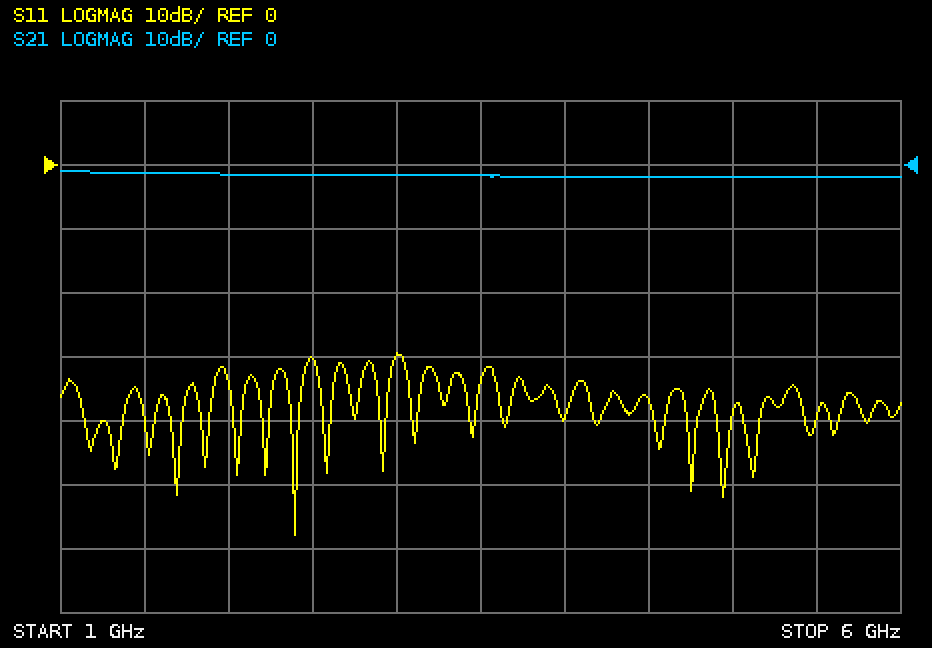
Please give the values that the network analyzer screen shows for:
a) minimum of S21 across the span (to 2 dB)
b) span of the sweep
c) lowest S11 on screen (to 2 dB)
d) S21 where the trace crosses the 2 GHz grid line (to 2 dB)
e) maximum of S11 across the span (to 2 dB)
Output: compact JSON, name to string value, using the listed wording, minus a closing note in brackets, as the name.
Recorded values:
{"minimum of S21 across the span": "-2 dB", "span of the sweep": "5 GHz", "lowest S11 on screen": "-58 dB", "S21 where the trace crosses the 2 GHz grid line": "-2 dB", "maximum of S11 across the span": "-30 dB"}
